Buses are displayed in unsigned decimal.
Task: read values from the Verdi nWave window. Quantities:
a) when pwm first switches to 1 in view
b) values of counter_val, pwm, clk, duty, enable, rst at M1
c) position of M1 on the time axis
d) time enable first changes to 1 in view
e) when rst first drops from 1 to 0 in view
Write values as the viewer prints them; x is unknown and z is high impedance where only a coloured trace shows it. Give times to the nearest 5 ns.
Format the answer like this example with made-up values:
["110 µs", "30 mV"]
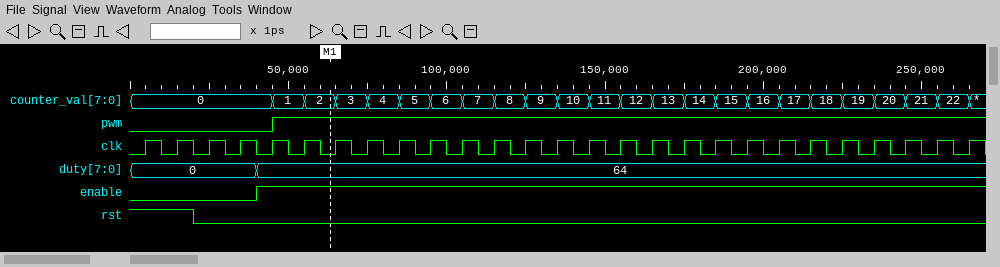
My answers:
["45 ns", "counter_val=2, pwm=1, clk=0, duty=64, enable=1, rst=0", "65 ns", "40 ns", "20 ns"]
